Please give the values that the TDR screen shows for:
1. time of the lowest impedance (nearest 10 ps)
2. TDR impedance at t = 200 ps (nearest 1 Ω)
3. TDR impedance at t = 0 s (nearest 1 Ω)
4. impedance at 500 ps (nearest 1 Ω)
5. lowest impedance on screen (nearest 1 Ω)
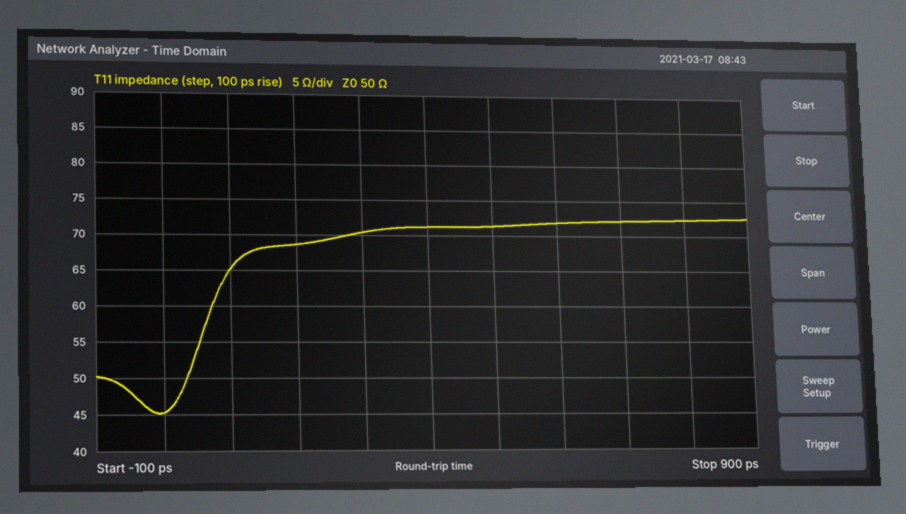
-10 ps
69 Ω
45 Ω
71 Ω
45 Ω
